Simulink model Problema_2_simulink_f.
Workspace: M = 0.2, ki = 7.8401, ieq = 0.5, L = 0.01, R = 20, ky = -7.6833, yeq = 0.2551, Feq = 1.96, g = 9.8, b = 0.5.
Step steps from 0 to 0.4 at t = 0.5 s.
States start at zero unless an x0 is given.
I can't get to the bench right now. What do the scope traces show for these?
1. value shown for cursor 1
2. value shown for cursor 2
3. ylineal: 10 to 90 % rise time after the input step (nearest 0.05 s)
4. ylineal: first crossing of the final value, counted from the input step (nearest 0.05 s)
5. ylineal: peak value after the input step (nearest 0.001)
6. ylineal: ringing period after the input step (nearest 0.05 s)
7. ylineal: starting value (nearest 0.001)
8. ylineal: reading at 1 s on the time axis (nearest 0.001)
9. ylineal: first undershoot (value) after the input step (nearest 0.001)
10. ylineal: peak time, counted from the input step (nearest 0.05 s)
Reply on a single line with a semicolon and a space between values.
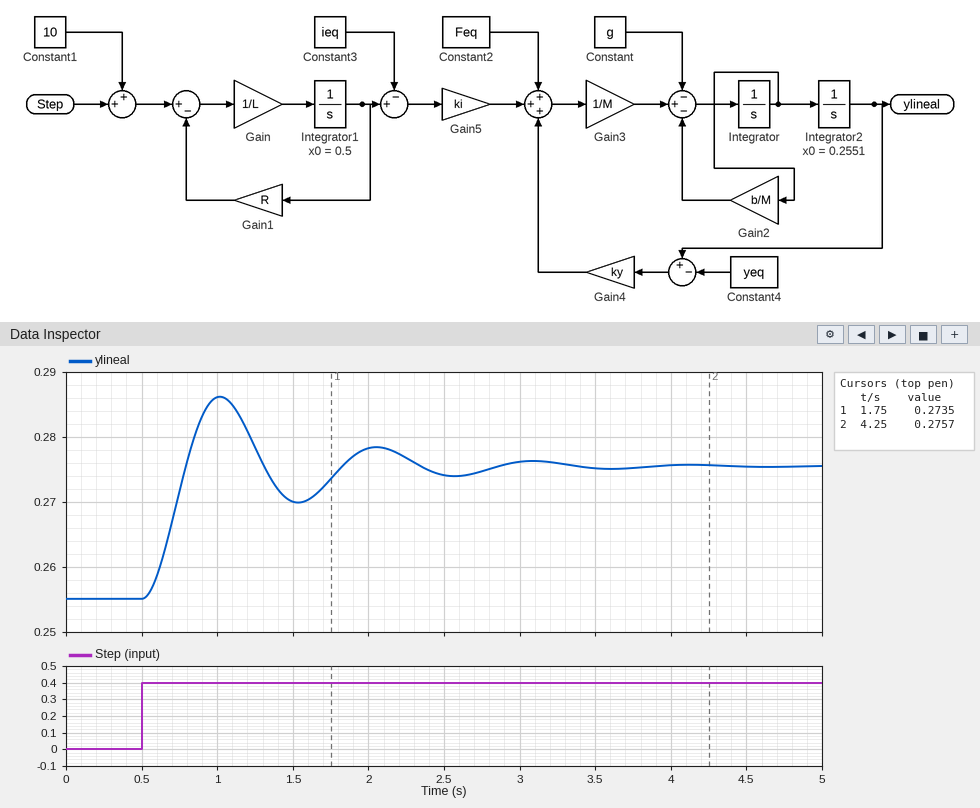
0.2735; 0.2757; 0.20 s; 0.30 s; 0.286; 1.05 s; 0.255; 0.286; 0.270; 0.50 s
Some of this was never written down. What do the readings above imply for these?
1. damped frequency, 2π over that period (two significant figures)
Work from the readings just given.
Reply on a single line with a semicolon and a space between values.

6.0 rad/s
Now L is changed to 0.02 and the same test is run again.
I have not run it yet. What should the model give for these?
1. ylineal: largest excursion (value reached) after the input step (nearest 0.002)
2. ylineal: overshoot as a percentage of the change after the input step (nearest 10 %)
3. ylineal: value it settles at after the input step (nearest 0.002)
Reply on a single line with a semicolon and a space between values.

0.286; 50 %; 0.276
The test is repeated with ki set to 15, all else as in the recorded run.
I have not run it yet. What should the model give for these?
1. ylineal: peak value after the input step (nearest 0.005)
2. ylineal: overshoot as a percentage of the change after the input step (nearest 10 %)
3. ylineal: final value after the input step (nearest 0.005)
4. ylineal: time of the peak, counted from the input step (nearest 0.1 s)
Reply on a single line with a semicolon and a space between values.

0.315; 50 %; 0.295; 0.5 s
